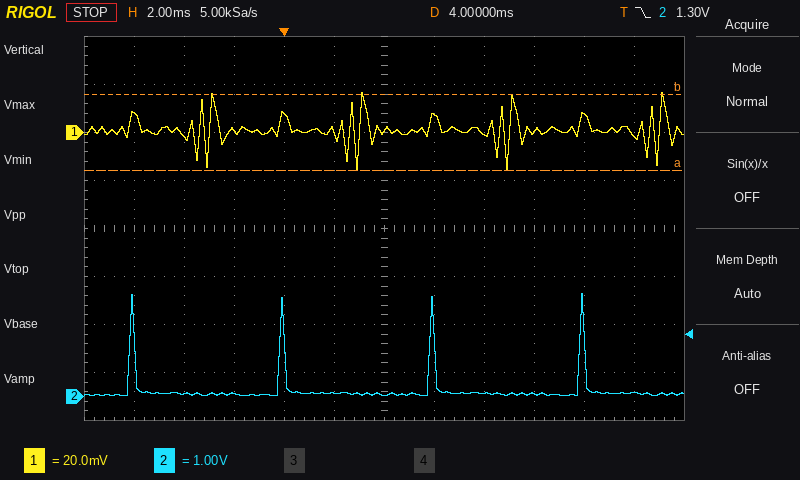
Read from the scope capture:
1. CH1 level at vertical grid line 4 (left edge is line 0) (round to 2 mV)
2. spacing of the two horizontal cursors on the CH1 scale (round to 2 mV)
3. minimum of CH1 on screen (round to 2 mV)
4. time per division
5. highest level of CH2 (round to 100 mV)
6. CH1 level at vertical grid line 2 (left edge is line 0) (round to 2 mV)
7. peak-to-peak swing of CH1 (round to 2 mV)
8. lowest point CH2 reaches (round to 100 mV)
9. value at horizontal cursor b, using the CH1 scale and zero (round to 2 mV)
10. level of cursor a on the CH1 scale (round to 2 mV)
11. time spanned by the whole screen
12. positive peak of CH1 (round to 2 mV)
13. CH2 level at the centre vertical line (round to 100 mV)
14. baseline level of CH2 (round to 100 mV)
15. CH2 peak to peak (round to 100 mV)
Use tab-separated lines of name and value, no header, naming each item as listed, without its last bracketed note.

CH1 level at vertical grid line 4 (left edge is line 0)	8 mV
spacing of the two horizontal cursors on the CH1 scale	32 mV
minimum of CH1 on screen	-16 mV
time per division	2 ms
highest level of CH2	2.1 V
CH1 level at vertical grid line 2 (left edge is line 0)	-2 mV
peak-to-peak swing of CH1	32 mV
lowest point CH2 reaches	0.0 V
value at horizontal cursor b, using the CH1 scale and zero	16 mV
level of cursor a on the CH1 scale	-16 mV
time spanned by the whole screen	24 ms
positive peak of CH1	16 mV
CH2 level at the centre vertical line	0.0 V
baseline level of CH2	100 mV
CH2 peak to peak	2.1 V
